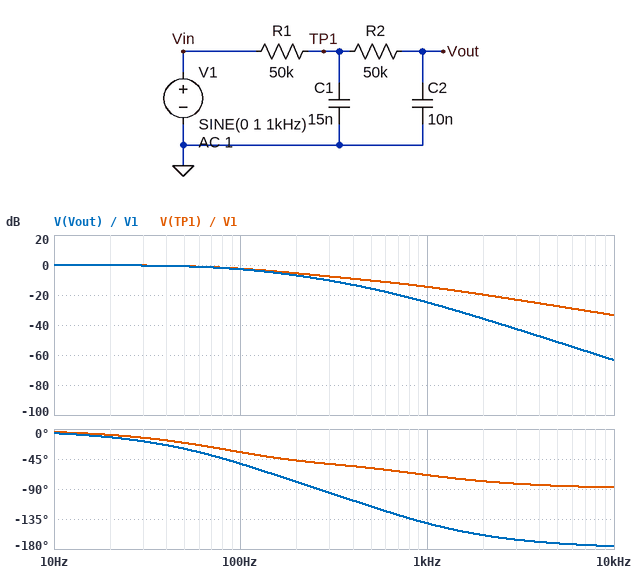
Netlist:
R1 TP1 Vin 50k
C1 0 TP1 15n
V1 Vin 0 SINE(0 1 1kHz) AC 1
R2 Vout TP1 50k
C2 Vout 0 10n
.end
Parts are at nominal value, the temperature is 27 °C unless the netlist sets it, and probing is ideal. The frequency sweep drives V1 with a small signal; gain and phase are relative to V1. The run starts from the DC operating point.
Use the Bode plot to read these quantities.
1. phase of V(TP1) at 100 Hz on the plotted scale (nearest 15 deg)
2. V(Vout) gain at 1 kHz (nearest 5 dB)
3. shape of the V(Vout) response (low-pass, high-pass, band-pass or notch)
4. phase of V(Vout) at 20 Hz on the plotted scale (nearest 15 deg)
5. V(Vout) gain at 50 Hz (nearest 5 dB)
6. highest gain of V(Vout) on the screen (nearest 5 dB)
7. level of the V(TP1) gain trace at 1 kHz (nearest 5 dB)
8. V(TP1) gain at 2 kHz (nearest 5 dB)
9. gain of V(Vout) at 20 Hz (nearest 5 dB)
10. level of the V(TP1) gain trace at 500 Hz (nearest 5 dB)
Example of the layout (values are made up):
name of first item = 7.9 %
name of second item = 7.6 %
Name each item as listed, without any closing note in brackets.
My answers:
phase of V(TP1) at 100 Hz on the plotted scale = -30 deg
V(Vout) gain at 1 kHz = -25 dB
shape of the V(Vout) response = low-pass
phase of V(Vout) at 20 Hz on the plotted scale = -15 deg
V(Vout) gain at 50 Hz = 0 dB
highest gain of V(Vout) on the screen = 0 dB
level of the V(TP1) gain trace at 1 kHz = -15 dB
V(TP1) gain at 2 kHz = -20 dB
gain of V(Vout) at 20 Hz = 0 dB
level of the V(TP1) gain trace at 500 Hz = -10 dB
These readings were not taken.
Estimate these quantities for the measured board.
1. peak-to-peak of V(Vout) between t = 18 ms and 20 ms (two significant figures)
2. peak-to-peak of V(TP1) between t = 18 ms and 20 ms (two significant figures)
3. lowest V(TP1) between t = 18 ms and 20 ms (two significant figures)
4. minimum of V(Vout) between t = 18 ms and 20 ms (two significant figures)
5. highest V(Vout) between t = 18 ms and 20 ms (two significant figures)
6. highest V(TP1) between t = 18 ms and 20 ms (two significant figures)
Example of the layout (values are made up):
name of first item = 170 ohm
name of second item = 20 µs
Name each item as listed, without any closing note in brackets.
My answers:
peak-to-peak of V(Vout) between t = 18 ms and 20 ms = 110 mV
peak-to-peak of V(TP1) between t = 18 ms and 20 ms = 370 mV
lowest V(TP1) between t = 18 ms and 20 ms = -190 mV
minimum of V(Vout) between t = 18 ms and 20 ms = -57 mV
highest V(Vout) between t = 18 ms and 20 ms = 57 mV
highest V(TP1) between t = 18 ms and 20 ms = 190 mV
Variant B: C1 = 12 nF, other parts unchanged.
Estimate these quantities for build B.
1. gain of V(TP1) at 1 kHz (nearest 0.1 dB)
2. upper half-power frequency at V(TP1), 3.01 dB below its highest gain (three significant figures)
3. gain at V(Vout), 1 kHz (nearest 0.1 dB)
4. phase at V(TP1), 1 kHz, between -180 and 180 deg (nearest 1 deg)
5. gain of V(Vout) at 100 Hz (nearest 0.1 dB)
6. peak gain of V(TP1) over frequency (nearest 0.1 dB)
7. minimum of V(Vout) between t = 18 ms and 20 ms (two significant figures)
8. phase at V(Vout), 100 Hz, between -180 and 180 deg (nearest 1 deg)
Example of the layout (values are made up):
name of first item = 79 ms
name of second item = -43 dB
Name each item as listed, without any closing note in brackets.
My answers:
gain of V(TP1) at 1 kHz = -13.0 dB
upper half-power frequency at V(TP1), 3.01 dB below its highest gain = 129 Hz
gain at V(Vout), 1 kHz = -23.4 dB
phase at V(TP1), 1 kHz, between -180 and 180 deg = -65 deg
gain of V(Vout) at 100 Hz = -2.5 dB
peak gain of V(TP1) over frequency = 0 dB
minimum of V(Vout) between t = 18 ms and 20 ms = -68 mV
phase at V(Vout), 100 Hz, between -180 and 180 deg = -49 deg
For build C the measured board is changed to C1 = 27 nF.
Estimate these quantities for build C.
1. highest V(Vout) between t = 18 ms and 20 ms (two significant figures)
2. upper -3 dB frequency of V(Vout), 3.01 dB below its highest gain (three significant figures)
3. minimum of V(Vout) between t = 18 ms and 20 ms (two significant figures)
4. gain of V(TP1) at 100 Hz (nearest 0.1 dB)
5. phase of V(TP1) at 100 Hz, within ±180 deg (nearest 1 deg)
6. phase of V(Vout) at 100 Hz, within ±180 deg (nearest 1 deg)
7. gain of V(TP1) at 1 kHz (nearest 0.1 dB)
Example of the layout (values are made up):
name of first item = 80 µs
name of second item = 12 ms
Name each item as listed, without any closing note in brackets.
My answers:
highest V(Vout) between t = 18 ms and 20 ms = 34 mV
upper -3 dB frequency of V(Vout), 3.01 dB below its highest gain = 76.9 Hz
minimum of V(Vout) between t = 18 ms and 20 ms = -34 mV
gain of V(TP1) at 100 Hz = -3.9 dB
phase of V(TP1) at 100 Hz, within ±180 deg = -46 deg
phase of V(Vout) at 100 Hz, within ±180 deg = -64 deg
gain of V(TP1) at 1 kHz = -19.1 dB
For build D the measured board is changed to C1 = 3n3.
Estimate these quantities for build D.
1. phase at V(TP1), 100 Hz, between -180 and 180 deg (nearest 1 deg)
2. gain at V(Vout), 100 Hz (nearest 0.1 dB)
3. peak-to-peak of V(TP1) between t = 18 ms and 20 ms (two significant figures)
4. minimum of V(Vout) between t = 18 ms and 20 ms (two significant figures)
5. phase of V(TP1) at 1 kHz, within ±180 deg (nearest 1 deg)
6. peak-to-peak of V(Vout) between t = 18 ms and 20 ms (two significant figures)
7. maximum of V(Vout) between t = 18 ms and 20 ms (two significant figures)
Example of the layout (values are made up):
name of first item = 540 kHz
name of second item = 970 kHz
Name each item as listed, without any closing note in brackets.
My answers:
phase at V(TP1), 100 Hz, between -180 and 180 deg = -20 deg
gain at V(Vout), 100 Hz = -1.7 dB
peak-to-peak of V(TP1) between t = 18 ms and 20 ms = 860 mV
minimum of V(Vout) between t = 18 ms and 20 ms = -130 mV
phase of V(TP1) at 1 kHz, within ±180 deg = -35 deg
peak-to-peak of V(Vout) between t = 18 ms and 20 ms = 260 mV
maximum of V(Vout) between t = 18 ms and 20 ms = 130 mV
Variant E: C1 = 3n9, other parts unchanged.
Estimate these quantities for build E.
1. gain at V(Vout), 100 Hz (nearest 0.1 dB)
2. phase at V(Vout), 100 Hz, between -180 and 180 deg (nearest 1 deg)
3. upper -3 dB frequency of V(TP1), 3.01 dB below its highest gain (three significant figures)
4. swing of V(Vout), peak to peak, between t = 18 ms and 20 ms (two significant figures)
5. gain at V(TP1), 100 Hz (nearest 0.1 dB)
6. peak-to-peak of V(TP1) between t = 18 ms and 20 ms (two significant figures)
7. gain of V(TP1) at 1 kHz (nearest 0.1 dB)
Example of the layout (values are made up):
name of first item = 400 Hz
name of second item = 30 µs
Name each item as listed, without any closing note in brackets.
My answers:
gain at V(Vout), 100 Hz = -1.7 dB
phase at V(Vout), 100 Hz, between -180 and 180 deg = -38 deg
upper -3 dB frequency of V(TP1), 3.01 dB below its highest gain = 184 Hz
swing of V(Vout), peak to peak, between t = 18 ms and 20 ms = 250 mV
gain at V(TP1), 100 Hz = -1.3 dB
peak-to-peak of V(TP1) between t = 18 ms and 20 ms = 820 mV
gain of V(TP1) at 1 kHz = -7.7 dB
